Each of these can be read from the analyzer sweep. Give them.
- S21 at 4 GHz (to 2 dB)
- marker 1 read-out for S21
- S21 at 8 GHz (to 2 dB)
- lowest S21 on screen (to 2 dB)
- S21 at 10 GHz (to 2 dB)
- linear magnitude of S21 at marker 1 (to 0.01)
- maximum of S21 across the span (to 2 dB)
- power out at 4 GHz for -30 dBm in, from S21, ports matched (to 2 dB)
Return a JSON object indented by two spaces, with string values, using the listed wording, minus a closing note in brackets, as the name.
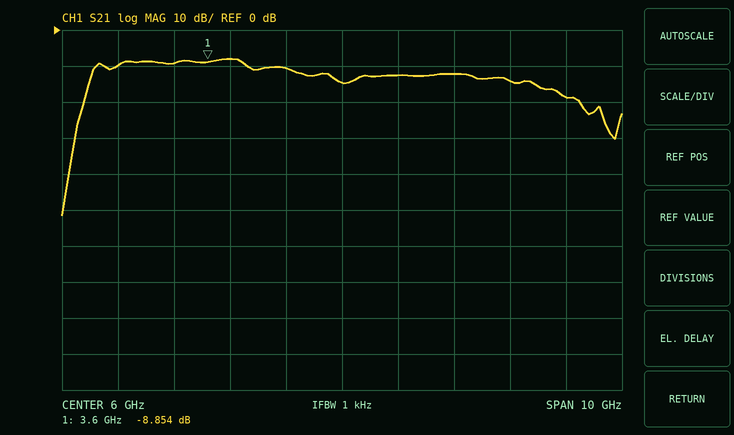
{
  "S21 at 4 GHz": "-8 dB",
  "marker 1 read-out for S21": "-8.854 dB",
  "S21 at 8 GHz": "-12 dB",
  "lowest S21 on screen": "-52 dB",
  "S21 at 10 GHz": "-18 dB",
  "linear magnitude of S21 at marker 1": "0.36",
  "maximum of S21 across the span": "-8 dB",
  "power out at 4 GHz for -30 dBm in, from S21, ports matched": "-38 dBm"
}
